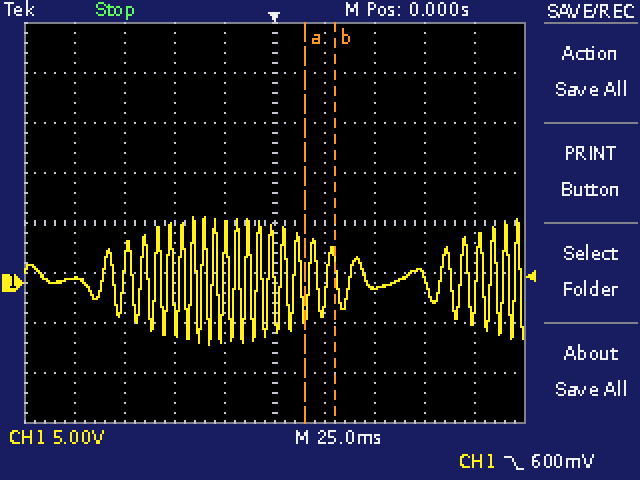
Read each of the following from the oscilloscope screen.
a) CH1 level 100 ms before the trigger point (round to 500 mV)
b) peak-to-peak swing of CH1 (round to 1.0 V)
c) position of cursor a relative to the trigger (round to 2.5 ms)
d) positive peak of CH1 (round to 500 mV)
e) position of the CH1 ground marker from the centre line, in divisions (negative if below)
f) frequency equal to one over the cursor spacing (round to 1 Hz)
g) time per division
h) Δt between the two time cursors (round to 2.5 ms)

500 mV
13.0 V
+15.0 ms
6.5 V
-1.2 div
67 Hz
25 ms
15.0 ms
